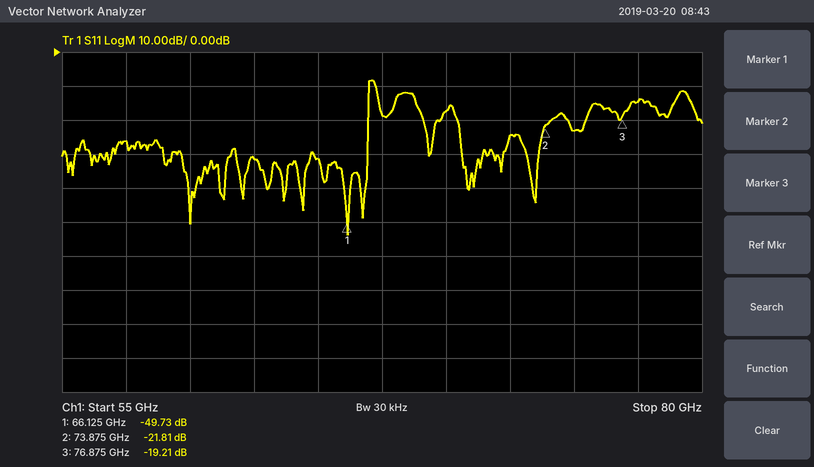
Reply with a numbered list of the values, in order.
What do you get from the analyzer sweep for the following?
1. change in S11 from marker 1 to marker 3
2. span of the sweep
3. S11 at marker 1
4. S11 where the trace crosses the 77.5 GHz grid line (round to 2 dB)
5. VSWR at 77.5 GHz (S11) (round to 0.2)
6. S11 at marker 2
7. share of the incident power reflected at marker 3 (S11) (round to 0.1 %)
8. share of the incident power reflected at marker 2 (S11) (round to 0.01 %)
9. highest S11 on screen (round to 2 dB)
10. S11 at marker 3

1. 30.52 dB
2. 25 GHz
3. -49.73 dB
4. -14 dB
5. 1.4
6. -21.81 dB
7. 1.2 %
8. 0.66 %
9. -8 dB
10. -19.21 dB
